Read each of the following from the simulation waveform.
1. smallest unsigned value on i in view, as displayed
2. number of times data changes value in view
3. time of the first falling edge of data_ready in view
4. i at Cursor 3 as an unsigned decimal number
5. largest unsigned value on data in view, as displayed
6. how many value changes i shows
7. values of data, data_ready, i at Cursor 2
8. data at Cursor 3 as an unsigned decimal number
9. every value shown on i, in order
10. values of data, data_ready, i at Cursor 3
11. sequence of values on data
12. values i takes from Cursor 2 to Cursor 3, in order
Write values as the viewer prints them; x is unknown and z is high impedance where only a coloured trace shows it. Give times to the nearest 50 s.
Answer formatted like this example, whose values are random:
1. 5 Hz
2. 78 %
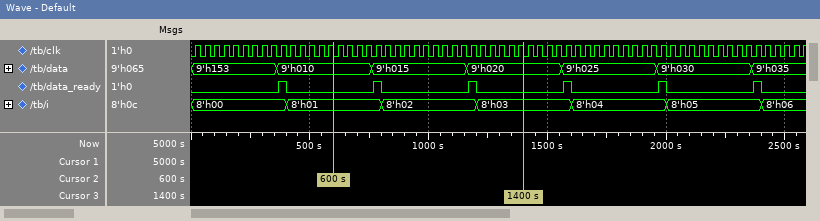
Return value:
1. 8'h00
2. 6
3. 400 s
4. 3
5. 9'h153
6. 6
7. data=9'h010, data_ready=0, i=8'h01
8. 32
9. 8'h00, 8'h01, 8'h02, 8'h03, 8'h04, 8'h05, 8'h06
10. data=9'h020, data_ready=0, i=8'h03
11. 9'h153, 9'h010, 9'h015, 9'h020, 9'h025, 9'h030, 9'h035
12. 8'h01, 8'h02, 8'h03
